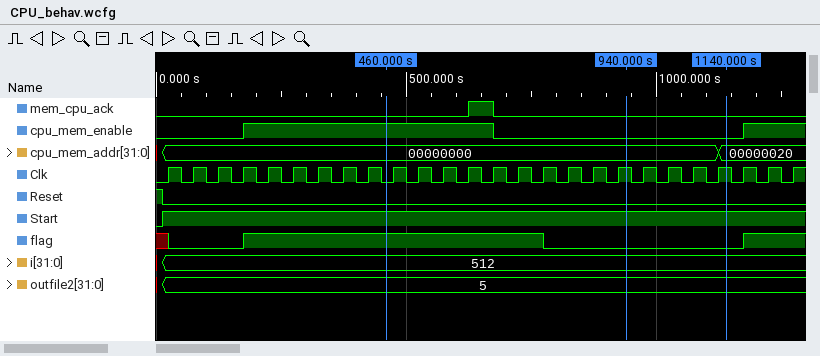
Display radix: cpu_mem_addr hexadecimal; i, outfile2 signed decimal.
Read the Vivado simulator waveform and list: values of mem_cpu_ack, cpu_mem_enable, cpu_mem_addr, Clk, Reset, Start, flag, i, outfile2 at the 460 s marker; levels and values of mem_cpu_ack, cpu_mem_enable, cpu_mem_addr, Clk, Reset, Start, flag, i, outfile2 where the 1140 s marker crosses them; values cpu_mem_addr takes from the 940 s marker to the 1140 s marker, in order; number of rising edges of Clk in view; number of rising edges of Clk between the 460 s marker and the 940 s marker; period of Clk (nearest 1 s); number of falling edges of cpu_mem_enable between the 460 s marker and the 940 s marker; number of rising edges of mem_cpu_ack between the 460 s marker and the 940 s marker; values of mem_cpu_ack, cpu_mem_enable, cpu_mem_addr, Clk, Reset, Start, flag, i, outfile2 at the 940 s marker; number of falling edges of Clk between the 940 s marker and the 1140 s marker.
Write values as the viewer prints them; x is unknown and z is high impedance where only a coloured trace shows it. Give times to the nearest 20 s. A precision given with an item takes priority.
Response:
mem_cpu_ack=0, cpu_mem_enable=1, cpu_mem_addr=00000000, Clk=0, Reset=0, Start=1, flag=1, i=512, outfile2=5
mem_cpu_ack=0, cpu_mem_enable=0, cpu_mem_addr=00000020, Clk=1, Reset=0, Start=1, flag=0, i=512, outfile2=5
00000000, 00000020
26
10
50 s
1
1
mem_cpu_ack=0, cpu_mem_enable=0, cpu_mem_addr=00000000, Clk=1, Reset=0, Start=1, flag=0, i=512, outfile2=5
4
